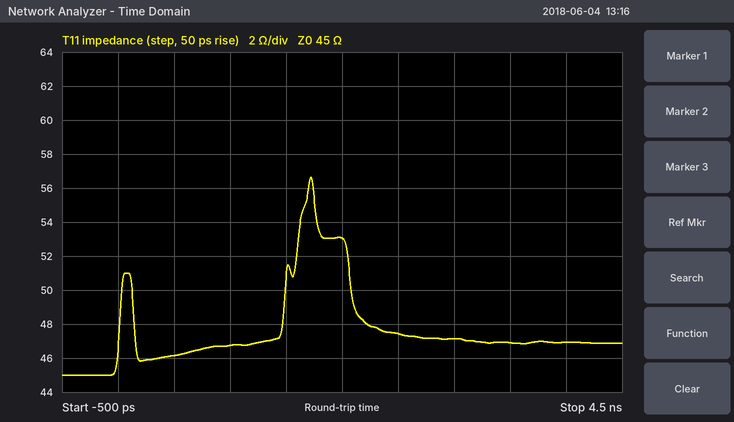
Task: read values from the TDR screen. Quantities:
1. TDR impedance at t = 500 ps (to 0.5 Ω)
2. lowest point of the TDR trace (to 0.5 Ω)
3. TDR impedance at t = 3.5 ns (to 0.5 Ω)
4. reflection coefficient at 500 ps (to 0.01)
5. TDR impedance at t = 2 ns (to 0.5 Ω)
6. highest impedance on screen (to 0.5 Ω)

46.0 Ω
45.0 Ω
47.0 Ω
+0.01
53.0 Ω
56.5 Ω
